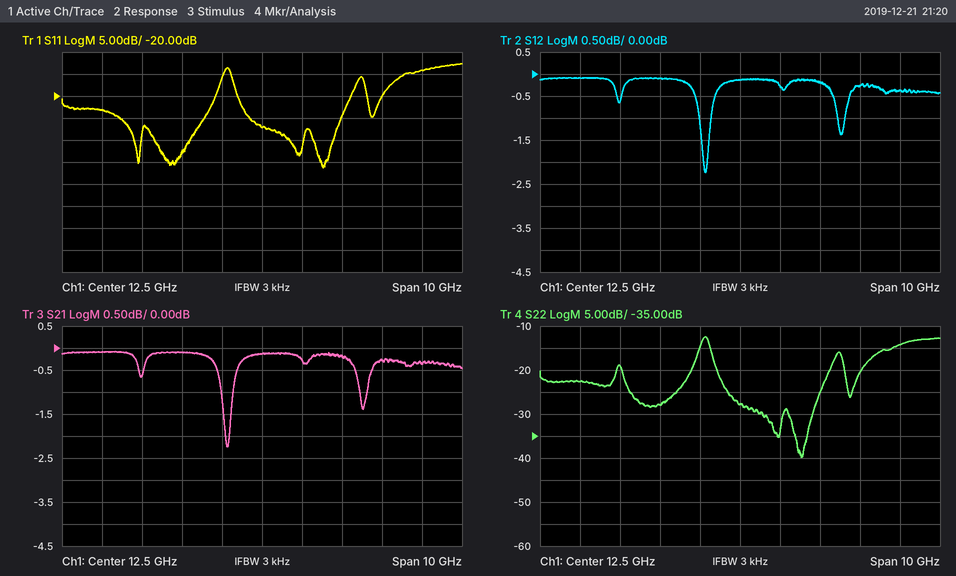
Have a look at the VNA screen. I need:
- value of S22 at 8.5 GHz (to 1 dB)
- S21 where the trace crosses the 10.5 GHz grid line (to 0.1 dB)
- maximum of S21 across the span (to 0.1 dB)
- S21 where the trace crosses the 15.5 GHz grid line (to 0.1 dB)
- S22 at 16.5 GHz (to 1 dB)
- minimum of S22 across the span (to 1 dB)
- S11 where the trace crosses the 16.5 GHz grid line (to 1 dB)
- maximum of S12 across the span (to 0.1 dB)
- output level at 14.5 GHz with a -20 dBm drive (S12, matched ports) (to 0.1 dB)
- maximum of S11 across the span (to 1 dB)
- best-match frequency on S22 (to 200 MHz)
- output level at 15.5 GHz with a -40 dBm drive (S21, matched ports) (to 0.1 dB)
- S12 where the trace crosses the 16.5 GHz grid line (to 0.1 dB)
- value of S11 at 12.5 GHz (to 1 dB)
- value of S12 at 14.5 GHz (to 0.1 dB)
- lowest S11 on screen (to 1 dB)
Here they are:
-23 dB
-0.1 dB
-0.1 dB
-0.3 dB
-14 dB
-40 dB
-14 dB
-0.1 dB
-20.2 dBm
-13 dB
14.0 GHz
-40.3 dBm
-0.4 dB
-27 dB
-0.2 dB
-36 dB
